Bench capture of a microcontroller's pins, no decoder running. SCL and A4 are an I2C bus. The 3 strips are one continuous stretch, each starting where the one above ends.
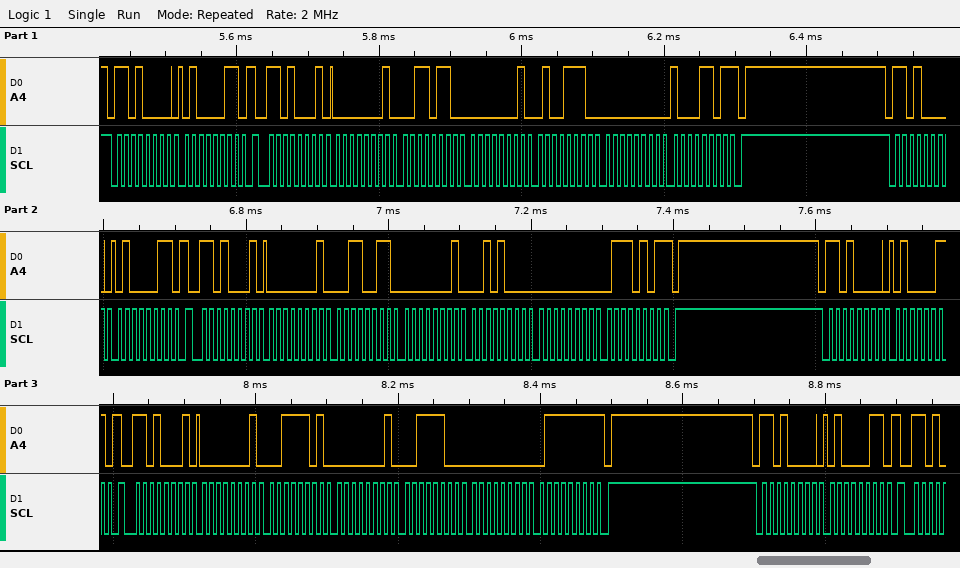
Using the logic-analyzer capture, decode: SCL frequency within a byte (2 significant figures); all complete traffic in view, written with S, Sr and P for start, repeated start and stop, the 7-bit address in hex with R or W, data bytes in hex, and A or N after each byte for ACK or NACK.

100 kHz
S 68W A 43 A Sr 68R A 01 A 36 A 01 A 4E A 00 A 8D N P S 68W A 43 A Sr 68R A 01 A 33 A 01 A 28 A 00 A 75 N P S 68W A 43 A Sr 68R A 01 A 3D A 01 A 3C A 00 A 7F N P S 68W A 43 A
